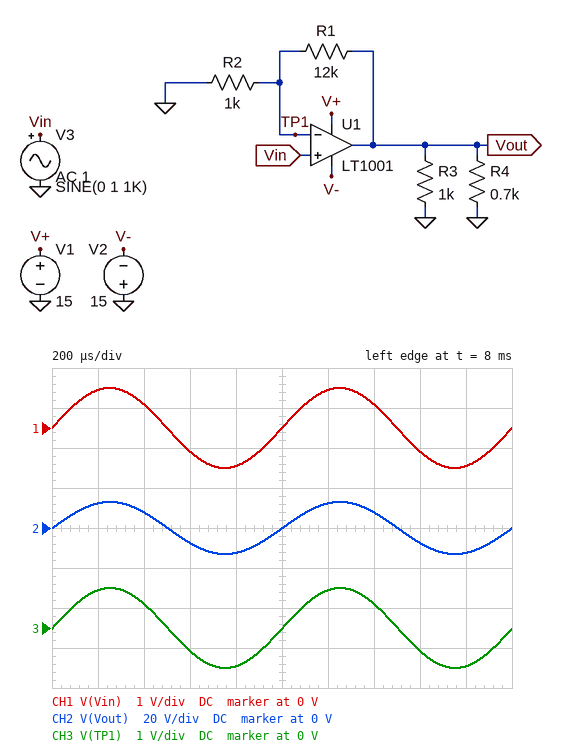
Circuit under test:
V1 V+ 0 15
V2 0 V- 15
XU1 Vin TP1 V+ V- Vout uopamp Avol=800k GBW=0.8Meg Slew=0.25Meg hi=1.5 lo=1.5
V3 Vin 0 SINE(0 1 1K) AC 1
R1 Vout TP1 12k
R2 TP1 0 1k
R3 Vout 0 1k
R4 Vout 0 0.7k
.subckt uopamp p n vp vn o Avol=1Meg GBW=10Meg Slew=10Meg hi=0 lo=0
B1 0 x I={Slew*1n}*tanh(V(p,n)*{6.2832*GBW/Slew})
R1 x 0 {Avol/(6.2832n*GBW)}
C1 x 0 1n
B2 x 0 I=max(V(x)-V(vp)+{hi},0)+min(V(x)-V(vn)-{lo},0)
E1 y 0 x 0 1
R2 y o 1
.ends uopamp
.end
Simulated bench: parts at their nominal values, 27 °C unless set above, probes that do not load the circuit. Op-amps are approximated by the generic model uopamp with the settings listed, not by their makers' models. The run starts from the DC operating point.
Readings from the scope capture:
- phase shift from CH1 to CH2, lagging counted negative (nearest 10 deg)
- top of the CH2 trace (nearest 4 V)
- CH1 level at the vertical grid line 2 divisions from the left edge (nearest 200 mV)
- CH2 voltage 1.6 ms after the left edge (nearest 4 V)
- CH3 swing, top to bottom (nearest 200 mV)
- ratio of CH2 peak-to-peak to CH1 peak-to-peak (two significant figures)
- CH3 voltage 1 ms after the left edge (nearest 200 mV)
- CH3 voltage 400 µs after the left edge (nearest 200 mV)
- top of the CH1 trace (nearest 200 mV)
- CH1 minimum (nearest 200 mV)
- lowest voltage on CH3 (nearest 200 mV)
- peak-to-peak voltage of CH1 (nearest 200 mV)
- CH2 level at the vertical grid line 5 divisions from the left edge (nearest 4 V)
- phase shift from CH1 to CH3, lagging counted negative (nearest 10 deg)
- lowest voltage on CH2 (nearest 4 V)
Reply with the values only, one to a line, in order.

0 deg
12 V
600 mV
-8 V
2.0 V
13
0 V
600 mV
1.0 V
-1.0 V
-1.0 V
2.0 V
0 V
0 deg
-12 V
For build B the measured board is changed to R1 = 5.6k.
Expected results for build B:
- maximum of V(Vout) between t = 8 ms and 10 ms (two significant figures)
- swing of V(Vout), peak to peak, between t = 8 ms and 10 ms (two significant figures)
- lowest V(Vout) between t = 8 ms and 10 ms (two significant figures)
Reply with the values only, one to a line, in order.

6.6 V
13 V
-6.6 V
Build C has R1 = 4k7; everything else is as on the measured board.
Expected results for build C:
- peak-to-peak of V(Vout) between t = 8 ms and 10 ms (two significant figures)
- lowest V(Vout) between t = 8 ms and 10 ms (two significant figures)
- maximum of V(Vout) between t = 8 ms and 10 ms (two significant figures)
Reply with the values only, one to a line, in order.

11 V
-5.7 V
5.7 V
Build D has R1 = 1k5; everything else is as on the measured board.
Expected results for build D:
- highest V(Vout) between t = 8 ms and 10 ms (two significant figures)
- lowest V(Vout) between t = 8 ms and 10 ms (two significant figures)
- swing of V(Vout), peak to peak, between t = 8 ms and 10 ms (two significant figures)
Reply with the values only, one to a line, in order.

2.5 V
-2.5 V
5.0 V
